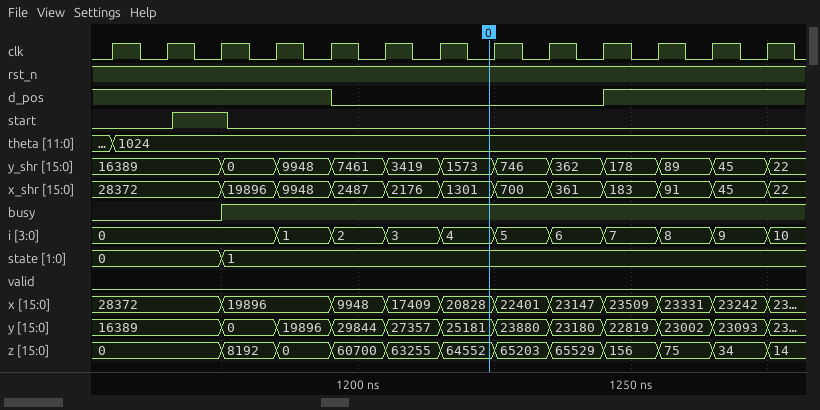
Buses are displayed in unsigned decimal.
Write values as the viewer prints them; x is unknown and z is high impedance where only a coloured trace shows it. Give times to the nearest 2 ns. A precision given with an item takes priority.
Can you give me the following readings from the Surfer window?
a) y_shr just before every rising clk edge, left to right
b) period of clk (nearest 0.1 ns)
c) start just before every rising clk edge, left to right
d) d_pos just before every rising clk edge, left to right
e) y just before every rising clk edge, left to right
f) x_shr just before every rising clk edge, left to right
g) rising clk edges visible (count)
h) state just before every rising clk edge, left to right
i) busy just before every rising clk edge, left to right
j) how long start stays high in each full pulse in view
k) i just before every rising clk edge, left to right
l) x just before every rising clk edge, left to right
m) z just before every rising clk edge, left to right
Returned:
16389, 16389, 16389, 0, 9948, 7461, 3419, 1573, 746, 362, 178, 89, 45
10 ns
0 0 1 0 0 0 0 0 0 0 0 0 0
1 1 1 1 1 0 0 0 0 0 1 1 1
16389, 16389, 16389, 0, 19896, 29844, 27357, 25181, 23880, 23180, 22819, 23002, 23093
28372, 28372, 28372, 19896, 9948, 2487, 2176, 1301, 700, 361, 183, 91, 45
13
0, 0, 0, 1, 1, 1, 1, 1, 1, 1, 1, 1, 1
0 0 0 1 1 1 1 1 1 1 1 1 1
10 ns
0, 0, 0, 0, 1, 2, 3, 4, 5, 6, 7, 8, 9
28372, 28372, 28372, 19896, 19896, 9948, 17409, 20828, 22401, 23147, 23509, 23331, 23242
0, 0, 0, 8192, 0, 60700, 63255, 64552, 65203, 65529, 156, 75, 34
